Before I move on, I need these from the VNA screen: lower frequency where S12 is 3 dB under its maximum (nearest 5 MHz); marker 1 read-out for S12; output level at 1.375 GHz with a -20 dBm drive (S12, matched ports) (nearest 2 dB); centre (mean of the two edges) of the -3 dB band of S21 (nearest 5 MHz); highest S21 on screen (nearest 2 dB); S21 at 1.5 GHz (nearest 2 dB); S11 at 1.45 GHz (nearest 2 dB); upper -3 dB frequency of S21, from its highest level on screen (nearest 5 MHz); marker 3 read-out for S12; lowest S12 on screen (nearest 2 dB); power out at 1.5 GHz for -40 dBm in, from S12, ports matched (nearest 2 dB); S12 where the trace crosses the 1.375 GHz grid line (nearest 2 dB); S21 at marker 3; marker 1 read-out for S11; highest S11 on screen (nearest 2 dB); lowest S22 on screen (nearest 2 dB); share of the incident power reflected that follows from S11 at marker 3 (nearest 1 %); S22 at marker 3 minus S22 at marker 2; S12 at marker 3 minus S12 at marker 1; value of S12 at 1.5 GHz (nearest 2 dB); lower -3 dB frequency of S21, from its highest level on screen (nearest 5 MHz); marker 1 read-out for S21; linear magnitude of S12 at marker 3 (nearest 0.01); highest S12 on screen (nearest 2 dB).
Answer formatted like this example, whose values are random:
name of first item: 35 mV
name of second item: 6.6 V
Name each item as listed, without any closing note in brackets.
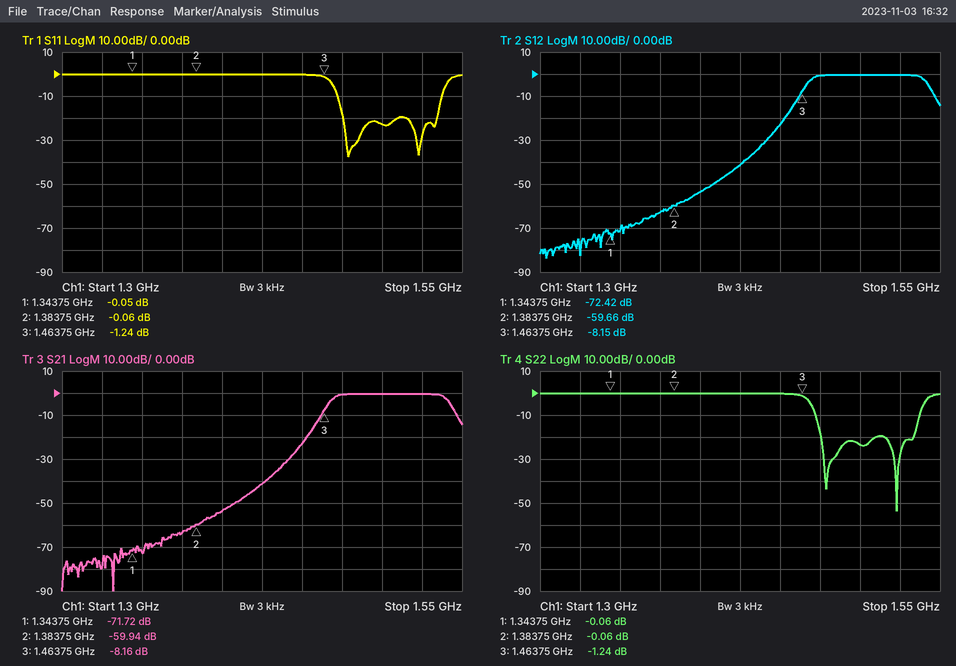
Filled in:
lower frequency where S12 is 3 dB under its maximum: 1.470 GHz
marker 1 read-out for S12: -72.42 dB
output level at 1.375 GHz with a -20 dBm drive (S12, matched ports): -82 dBm
centre (mean of the two edges) of the -3 dB band of S21: 1.505 GHz
highest S21 on screen: 0 dB
S21 at 1.5 GHz: 0 dB
S11 at 1.45 GHz: 0 dB
upper -3 dB frequency of S21, from its highest level on screen: 1.540 GHz
marker 3 read-out for S12: -8.15 dB
lowest S12 on screen: -84 dB
power out at 1.5 GHz for -40 dBm in, from S12, ports matched: -40 dBm
S12 where the trace crosses the 1.375 GHz grid line: -62 dB
S21 at marker 3: -8.16 dB
marker 1 read-out for S11: -0.05 dB
highest S11 on screen: 0 dB
lowest S22 on screen: -54 dB
share of the incident power reflected that follows from S11 at marker 3: 75 %
S22 at marker 3 minus S22 at marker 2: -1.18 dB
S12 at marker 3 minus S12 at marker 1: 64.27 dB
value of S12 at 1.5 GHz: 0 dB
lower -3 dB frequency of S21, from its highest level on screen: 1.470 GHz
marker 1 read-out for S21: -71.72 dB
linear magnitude of S12 at marker 3: 0.39
highest S12 on screen: 0 dB
